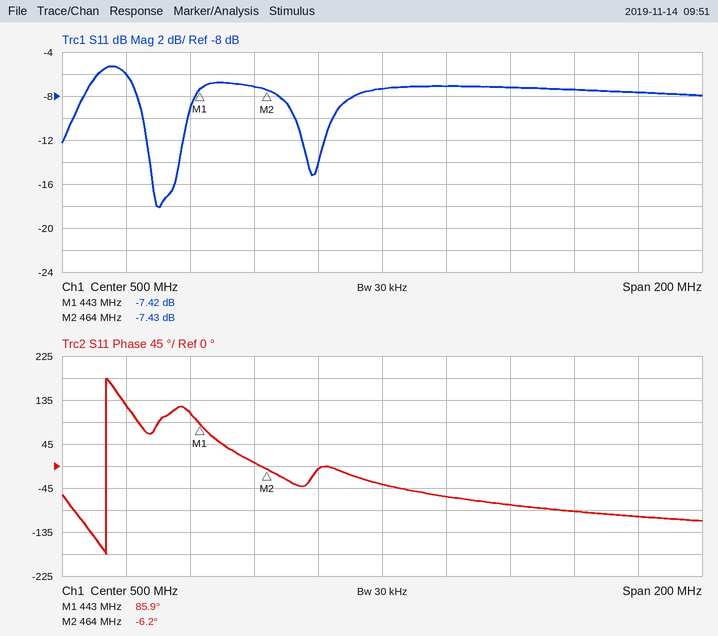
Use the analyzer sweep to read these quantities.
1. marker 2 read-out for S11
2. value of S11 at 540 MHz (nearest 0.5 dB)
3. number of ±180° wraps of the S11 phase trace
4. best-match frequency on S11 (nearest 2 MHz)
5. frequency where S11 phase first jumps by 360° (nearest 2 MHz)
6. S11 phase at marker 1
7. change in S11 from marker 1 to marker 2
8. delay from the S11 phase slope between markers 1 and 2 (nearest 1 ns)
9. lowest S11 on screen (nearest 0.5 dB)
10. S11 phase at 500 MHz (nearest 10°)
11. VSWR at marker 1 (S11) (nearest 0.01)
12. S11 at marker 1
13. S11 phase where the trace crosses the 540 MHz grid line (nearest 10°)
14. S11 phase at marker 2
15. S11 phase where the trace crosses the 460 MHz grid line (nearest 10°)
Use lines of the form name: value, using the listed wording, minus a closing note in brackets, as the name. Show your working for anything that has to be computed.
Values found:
marker 2 read-out for S11: -7.43 dB
value of S11 at 540 MHz: -7.0 dB
number of ±180° wraps of the S11 phase trace: 1
best-match frequency on S11: 430 MHz
frequency where S11 phase first jumps by 360°: 414 MHz
S11 phase at marker 1: 85.9°
change in S11 from marker 1 to marker 2: -7.43 − (-7.42) = -0.01 dB
delay from the S11 phase slope between markers 1 and 2: −(-6.2° − (85.9°))/(360° × 21 MHz) ≈ 12 ns
lowest S11 on screen: -18.0 dB
S11 phase at 500 MHz: -40°
VSWR at marker 1 (S11): (1 + 0.4256)/(1 − 0.4256) ≈ 2.48
S11 at marker 1: -7.42 dB
S11 phase where the trace crosses the 540 MHz grid line: -80°
S11 phase at marker 2: -6.2°
S11 phase where the trace crosses the 460 MHz grid line: 10°
